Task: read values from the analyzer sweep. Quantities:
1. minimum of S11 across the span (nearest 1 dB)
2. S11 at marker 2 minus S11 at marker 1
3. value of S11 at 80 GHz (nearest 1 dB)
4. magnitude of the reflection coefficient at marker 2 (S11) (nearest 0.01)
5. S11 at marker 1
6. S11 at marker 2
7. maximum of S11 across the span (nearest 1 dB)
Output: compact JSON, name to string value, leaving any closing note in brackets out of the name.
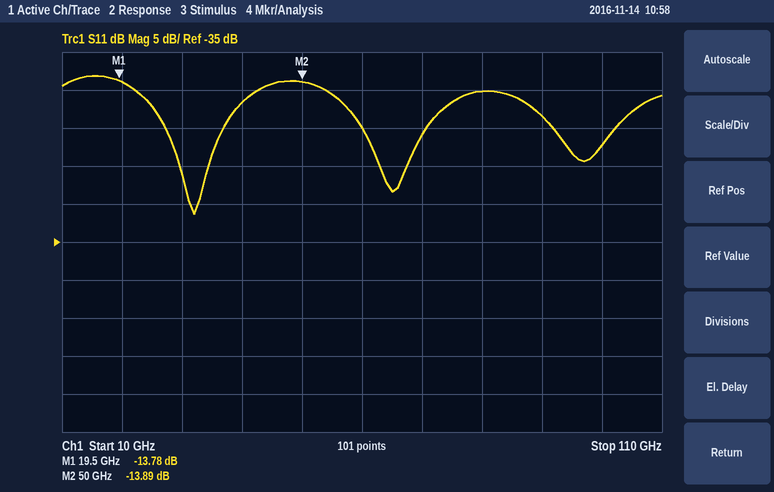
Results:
{"minimum of S11 across the span": "-31 dB", "S11 at marker 2 minus S11 at marker 1": "-0.11 dB", "value of S11 at 80 GHz": "-15 dB", "magnitude of the reflection coefficient at marker 2 (S11)": "0.20", "S11 at marker 1": "-13.78 dB", "S11 at marker 2": "-13.89 dB", "maximum of S11 across the span": "-13 dB"}
